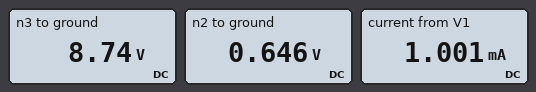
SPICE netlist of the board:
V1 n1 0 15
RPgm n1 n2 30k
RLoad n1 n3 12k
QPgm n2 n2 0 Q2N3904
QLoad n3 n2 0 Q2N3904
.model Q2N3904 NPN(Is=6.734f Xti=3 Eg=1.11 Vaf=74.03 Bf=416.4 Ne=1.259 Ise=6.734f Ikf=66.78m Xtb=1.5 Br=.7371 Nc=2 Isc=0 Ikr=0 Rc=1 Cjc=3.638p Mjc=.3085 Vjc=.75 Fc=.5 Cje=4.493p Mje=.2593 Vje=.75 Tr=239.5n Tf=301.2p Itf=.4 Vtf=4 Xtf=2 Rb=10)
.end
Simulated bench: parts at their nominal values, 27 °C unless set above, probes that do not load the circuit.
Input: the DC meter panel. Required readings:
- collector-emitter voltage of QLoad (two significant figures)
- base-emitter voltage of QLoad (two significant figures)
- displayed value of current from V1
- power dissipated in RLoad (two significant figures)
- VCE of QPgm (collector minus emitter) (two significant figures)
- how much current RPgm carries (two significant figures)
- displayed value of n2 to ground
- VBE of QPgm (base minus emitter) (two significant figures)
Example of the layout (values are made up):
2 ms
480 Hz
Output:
8.7 V
650 mV
1.001 mA
3.3 mW
650 mV
480 µA
0.646 V
650 mV
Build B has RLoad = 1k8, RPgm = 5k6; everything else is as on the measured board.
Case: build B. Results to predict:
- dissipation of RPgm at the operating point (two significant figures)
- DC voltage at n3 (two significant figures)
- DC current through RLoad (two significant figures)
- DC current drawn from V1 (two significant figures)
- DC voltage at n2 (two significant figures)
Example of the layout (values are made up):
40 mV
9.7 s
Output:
37 mW
9.9 V
2.8 mA
5.4 mA
690 mV
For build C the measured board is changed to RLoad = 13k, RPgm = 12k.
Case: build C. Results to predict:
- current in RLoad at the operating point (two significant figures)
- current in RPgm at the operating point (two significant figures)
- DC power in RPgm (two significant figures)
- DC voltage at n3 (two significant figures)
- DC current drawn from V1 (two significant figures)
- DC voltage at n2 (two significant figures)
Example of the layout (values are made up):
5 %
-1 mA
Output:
1.1 mA
1.2 mA
17 mW
140 mV
2.3 mA
670 mV
